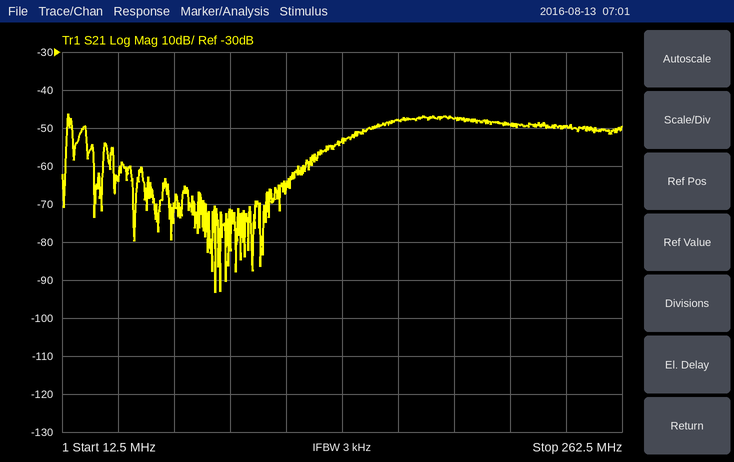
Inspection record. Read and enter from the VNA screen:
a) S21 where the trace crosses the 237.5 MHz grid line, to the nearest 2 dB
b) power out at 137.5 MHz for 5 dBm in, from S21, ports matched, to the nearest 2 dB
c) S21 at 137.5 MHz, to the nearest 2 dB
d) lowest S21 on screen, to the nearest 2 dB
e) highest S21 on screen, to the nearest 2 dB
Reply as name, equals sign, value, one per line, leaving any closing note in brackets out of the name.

S21 where the trace crosses the 237.5 MHz grid line, to the nearest 2 dB = -50 dB
power out at 137.5 MHz for 5 dBm in, from S21, ports matched, to the nearest 2 dB = -48 dBm
S21 at 137.5 MHz, to the nearest 2 dB = -54 dB
lowest S21 on screen, to the nearest 2 dB = -94 dB
highest S21 on screen, to the nearest 2 dB = -46 dB
